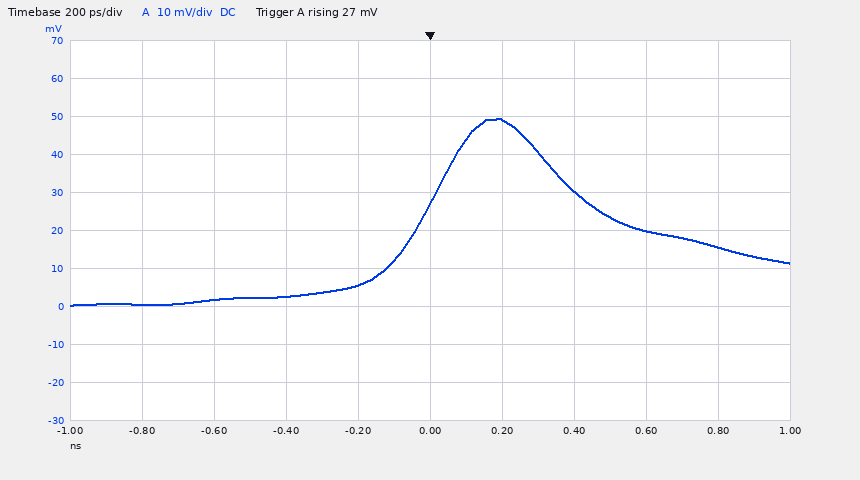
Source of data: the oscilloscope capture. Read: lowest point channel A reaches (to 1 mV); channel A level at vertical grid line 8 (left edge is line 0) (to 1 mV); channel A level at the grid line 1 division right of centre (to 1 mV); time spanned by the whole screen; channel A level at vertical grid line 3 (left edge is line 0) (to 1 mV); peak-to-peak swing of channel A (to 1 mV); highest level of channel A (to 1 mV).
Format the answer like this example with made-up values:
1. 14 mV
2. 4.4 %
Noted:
1. 0 mV
2. 20 mV
3. 49 mV
4. 2 ns
5. 3 mV
6. 49 mV
7. 49 mV
